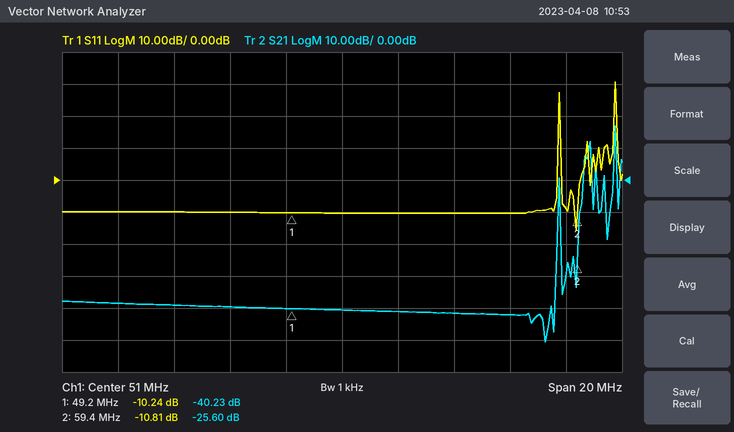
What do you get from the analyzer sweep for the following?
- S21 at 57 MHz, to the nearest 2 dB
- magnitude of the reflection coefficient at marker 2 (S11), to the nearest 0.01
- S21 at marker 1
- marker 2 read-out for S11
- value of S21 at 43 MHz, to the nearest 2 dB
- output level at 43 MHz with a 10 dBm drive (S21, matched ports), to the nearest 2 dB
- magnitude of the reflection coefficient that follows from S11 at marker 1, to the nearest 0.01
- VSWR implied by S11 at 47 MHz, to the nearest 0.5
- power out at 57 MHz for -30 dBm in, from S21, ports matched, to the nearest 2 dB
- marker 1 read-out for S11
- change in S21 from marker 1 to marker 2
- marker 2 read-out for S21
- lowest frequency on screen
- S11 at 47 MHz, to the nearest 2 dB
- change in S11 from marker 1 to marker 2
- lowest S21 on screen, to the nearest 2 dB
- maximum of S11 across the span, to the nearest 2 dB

-42 dB
0.29
-40.23 dB
-10.81 dB
-38 dB
-28 dBm
0.31
2.0
-72 dBm
-10.24 dB
14.63 dB
-25.60 dB
41 MHz
-10 dB
-0.57 dB
-50 dB
30 dB
